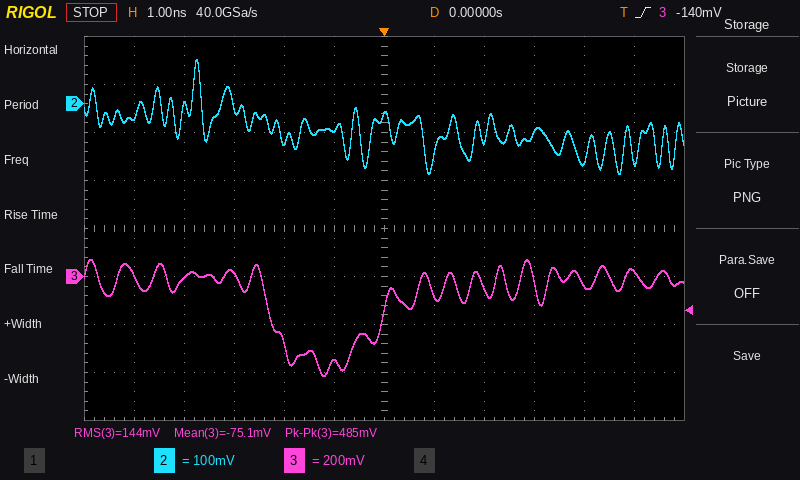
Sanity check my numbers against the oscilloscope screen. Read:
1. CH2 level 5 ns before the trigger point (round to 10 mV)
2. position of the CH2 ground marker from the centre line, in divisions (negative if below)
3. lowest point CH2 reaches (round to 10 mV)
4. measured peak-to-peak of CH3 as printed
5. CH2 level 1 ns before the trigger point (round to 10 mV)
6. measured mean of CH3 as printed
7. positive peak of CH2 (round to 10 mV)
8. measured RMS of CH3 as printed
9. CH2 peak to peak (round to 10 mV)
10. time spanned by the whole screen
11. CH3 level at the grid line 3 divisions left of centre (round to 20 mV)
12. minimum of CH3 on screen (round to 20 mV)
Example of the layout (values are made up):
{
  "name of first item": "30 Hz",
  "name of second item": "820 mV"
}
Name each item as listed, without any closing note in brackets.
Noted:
{
  "CH2 level 5 ns before the trigger point": "-20 mV",
  "position of the CH2 ground marker from the centre line, in divisions": "+2.6 div",
  "lowest point CH2 reaches": "-150 mV",
  "measured peak-to-peak of CH3 as printed": "485 mV",
  "CH2 level 1 ns before the trigger point": "-50 mV",
  "measured mean of CH3 as printed": "-75.1 mV",
  "positive peak of CH2": "90 mV",
  "measured RMS of CH3 as printed": "144 mV",
  "CH2 peak to peak": "240 mV",
  "time spanned by the whole screen": "12 ns",
  "CH3 level at the grid line 3 divisions left of centre": "20 mV",
  "minimum of CH3 on screen": "-420 mV"
}
